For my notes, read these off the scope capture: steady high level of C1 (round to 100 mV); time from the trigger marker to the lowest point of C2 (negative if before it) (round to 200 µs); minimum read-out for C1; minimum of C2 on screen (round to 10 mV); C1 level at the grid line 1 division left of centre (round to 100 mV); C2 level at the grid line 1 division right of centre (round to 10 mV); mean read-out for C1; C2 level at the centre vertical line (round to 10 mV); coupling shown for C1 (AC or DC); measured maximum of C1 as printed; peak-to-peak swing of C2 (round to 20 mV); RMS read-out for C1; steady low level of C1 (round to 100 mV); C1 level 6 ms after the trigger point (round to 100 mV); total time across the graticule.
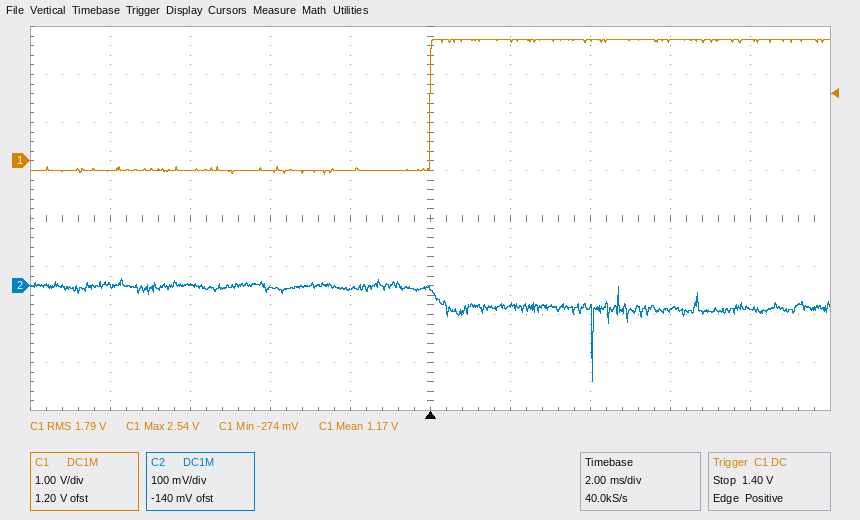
2.5 V
+4.0 ms
-274 mV
-200 mV
-200 mV
-40 mV
1.17 V
-10 mV
DC
2.54 V
220 mV
1.79 V
-200 mV
2.5 V
20 ms
